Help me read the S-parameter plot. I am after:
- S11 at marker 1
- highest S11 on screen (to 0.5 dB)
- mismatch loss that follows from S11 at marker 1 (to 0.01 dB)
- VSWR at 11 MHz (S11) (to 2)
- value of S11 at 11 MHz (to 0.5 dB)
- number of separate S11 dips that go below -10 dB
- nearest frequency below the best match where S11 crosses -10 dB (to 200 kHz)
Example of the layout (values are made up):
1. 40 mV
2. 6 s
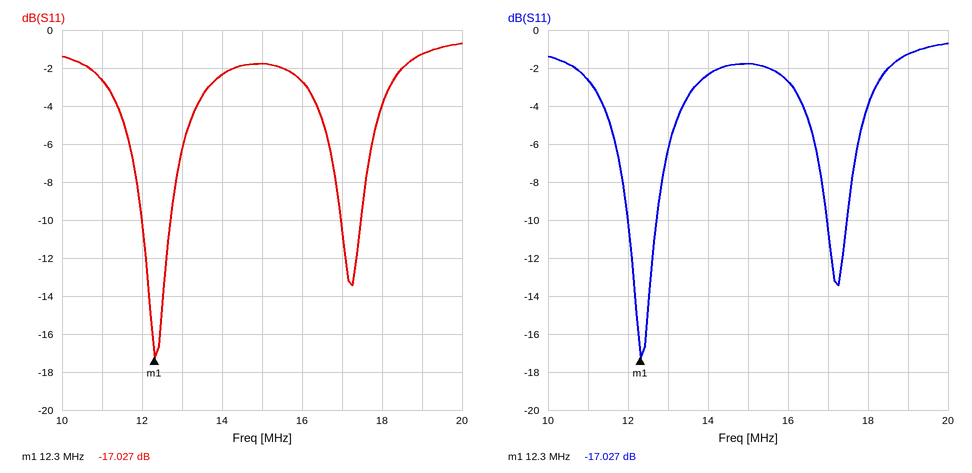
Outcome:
1. -17.027 dB
2. -0.5 dB
3. 0.09 dB
4. 6
5. -2.5 dB
6. 2
7. 12.0 MHz
